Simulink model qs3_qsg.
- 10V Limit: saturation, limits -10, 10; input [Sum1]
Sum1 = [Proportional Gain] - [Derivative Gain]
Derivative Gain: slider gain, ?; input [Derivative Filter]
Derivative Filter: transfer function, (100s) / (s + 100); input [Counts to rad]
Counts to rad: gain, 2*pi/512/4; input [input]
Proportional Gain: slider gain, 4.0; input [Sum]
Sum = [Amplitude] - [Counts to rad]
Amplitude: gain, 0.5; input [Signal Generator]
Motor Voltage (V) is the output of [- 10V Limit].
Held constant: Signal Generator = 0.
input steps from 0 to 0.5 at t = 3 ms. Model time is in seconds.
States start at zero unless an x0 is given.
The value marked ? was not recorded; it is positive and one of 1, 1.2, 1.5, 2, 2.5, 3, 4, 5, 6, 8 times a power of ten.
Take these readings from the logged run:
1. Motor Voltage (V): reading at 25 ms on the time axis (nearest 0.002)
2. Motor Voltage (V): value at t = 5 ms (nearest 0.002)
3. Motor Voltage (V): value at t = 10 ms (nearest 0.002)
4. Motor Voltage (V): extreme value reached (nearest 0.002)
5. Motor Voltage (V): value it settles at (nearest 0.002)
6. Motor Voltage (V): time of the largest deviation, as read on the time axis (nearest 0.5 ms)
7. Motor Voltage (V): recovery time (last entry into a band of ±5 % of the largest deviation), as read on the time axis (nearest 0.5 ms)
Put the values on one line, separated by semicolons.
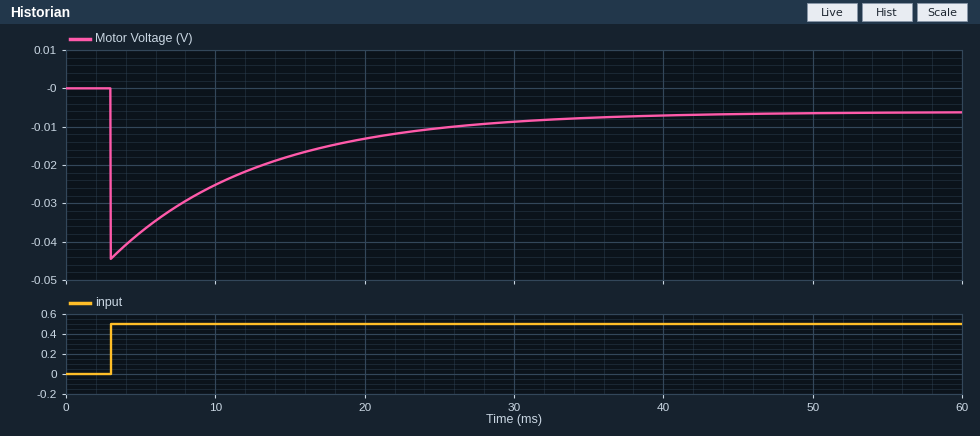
-0.010; -0.038; -0.026; -0.044; -0.006; 3.0 ms; 31.5 ms
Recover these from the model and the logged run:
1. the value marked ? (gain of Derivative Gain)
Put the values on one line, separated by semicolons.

0.25
